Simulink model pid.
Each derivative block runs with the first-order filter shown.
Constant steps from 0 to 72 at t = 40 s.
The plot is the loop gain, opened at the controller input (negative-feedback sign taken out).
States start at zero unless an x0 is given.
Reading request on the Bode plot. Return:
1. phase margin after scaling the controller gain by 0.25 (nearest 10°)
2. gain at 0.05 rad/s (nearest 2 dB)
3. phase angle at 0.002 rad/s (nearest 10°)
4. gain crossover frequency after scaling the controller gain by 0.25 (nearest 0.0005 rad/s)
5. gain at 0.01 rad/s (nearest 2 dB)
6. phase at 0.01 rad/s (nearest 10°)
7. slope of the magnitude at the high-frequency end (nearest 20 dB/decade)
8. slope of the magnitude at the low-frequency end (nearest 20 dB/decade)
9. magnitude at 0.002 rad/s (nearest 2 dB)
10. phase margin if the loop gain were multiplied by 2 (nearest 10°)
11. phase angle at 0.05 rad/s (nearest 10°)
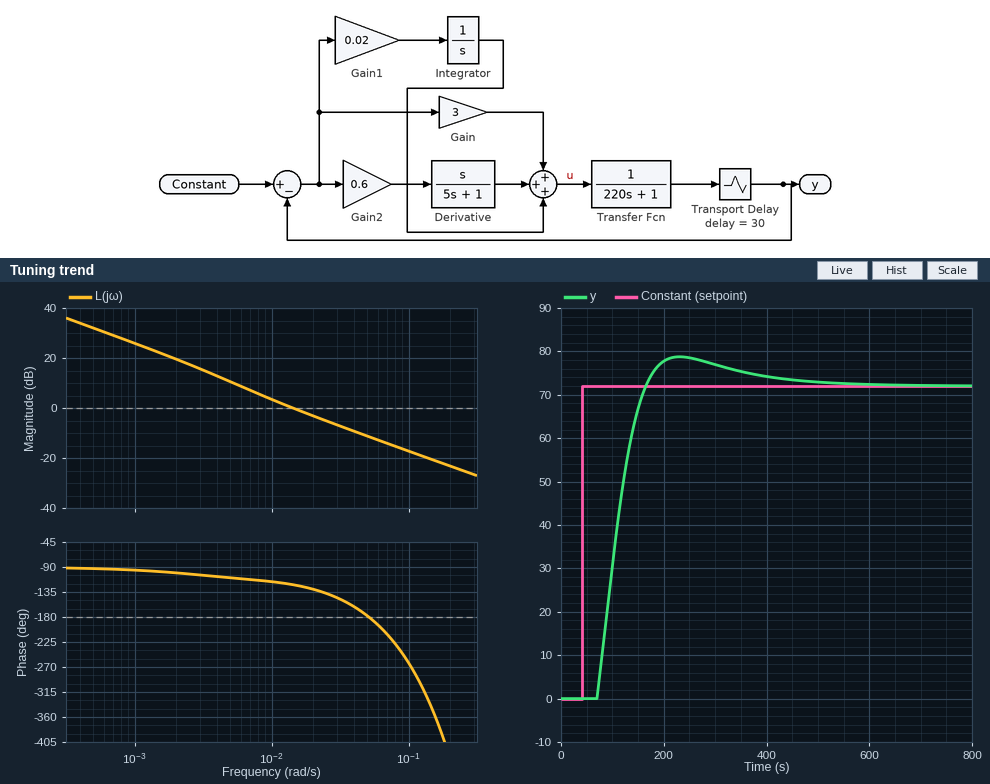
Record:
70°
-12 dB
-100°
0.0045 rad/s
4 dB
-120°
-20 dB/decade
-20 dB/decade
20 dB
40°
-180°
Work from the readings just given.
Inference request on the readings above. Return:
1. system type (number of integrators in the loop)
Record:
1
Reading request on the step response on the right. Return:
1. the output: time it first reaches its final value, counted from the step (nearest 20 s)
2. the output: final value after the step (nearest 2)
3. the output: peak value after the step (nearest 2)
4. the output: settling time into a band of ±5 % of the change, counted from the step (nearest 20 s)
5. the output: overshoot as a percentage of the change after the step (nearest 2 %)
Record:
120 s
72
78
300 s
10 %
